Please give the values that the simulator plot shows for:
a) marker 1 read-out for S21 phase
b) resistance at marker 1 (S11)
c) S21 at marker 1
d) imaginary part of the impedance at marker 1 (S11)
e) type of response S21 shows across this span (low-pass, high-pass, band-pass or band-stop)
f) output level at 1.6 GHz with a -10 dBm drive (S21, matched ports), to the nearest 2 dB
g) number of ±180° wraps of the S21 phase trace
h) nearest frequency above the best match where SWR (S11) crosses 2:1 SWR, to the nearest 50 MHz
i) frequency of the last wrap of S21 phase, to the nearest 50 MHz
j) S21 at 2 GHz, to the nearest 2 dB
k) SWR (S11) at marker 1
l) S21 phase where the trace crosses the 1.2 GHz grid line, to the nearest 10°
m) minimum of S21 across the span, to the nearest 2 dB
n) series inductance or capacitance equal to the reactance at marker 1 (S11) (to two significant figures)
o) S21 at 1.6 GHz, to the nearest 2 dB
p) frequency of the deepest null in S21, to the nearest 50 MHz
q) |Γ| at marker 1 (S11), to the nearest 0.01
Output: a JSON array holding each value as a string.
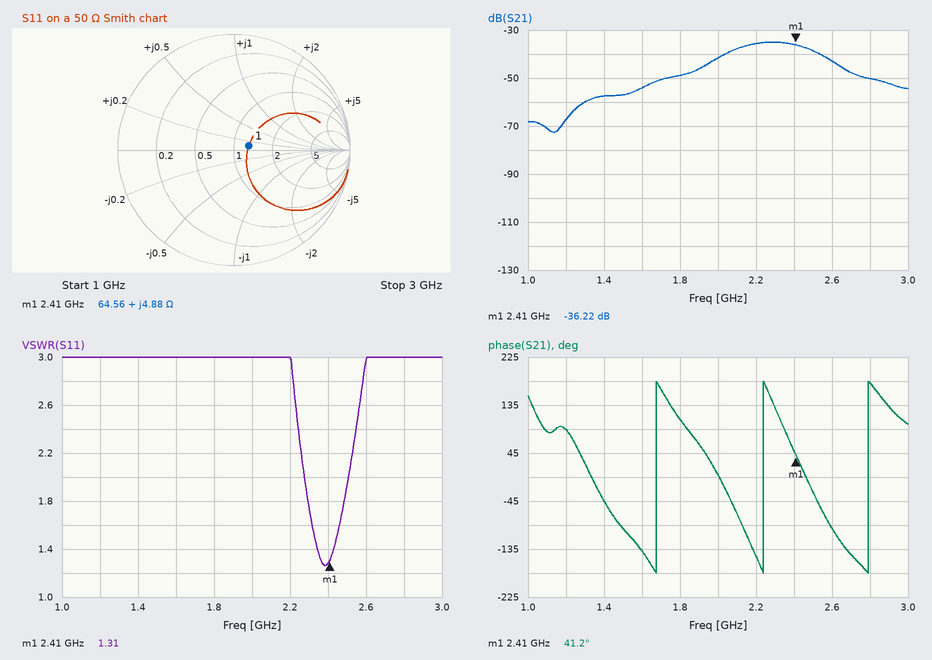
["41.2°", "64.56 Ω", "-36.22 dB", "+4.88 Ω", "band-pass", "-64 dBm", "3", "2.50 GHz", "2.80 GHz", "-42 dB", "1.31", "90°", "-72 dB", "320 pH", "-54 dB", "1.15 GHz", "0.13"]
